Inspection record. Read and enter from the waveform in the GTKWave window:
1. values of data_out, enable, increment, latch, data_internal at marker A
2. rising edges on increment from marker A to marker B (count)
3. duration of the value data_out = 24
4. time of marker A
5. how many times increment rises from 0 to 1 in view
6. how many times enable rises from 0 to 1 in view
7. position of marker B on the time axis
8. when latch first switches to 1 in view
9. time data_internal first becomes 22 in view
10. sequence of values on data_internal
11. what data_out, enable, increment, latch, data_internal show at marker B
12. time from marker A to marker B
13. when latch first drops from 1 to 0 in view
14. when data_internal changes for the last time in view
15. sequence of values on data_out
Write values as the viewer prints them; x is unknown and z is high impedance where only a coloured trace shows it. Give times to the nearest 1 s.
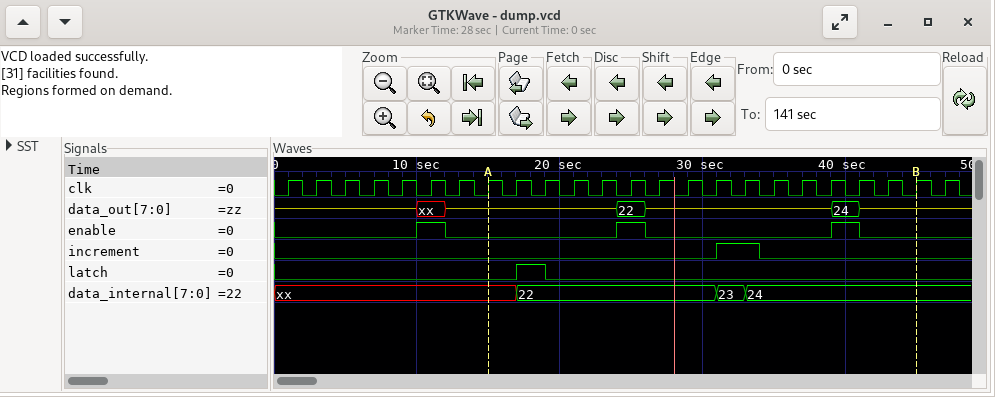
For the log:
data_out=z, enable=0, increment=0, latch=0, data_internal=xx
1
2 s
15 s
1
3
45 s
17 s
17 s
xx, 22, 23, 24
data_out=z, enable=0, increment=0, latch=0, data_internal=24
30 s
19 s
33 s
z, xx, z, 22, z, 24, z
